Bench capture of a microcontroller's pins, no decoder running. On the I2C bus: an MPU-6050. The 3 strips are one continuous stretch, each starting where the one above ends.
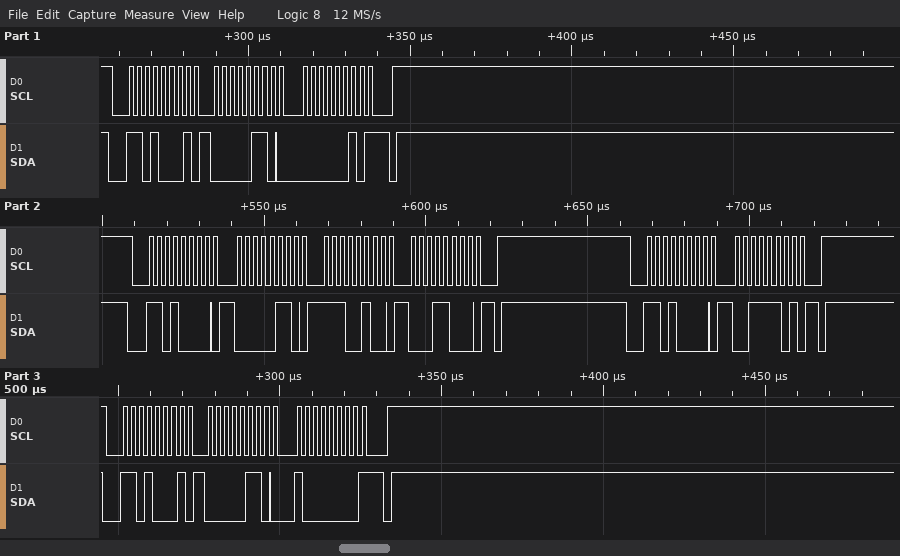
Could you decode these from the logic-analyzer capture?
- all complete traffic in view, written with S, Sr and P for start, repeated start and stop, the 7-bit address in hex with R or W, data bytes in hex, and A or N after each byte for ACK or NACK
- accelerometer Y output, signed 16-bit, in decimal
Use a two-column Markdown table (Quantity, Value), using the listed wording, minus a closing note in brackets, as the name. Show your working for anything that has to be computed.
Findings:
| Quantity | Value |
|---|---|
| all complete traffic in view, written with S, Sr and P for start, repeated start and stop, the 7-bit address in hex with R or W, data bytes in hex, and A or N after each byte for ACK or NACK | S 68R A 06 A 02 N P S 68W A 06 A E4 A 18 A P S 68W A 3D A P S 68R A 06 A 80 N P |
| accelerometer Y output, signed 16-bit, in decimal | 0x0680 = 1664 |
